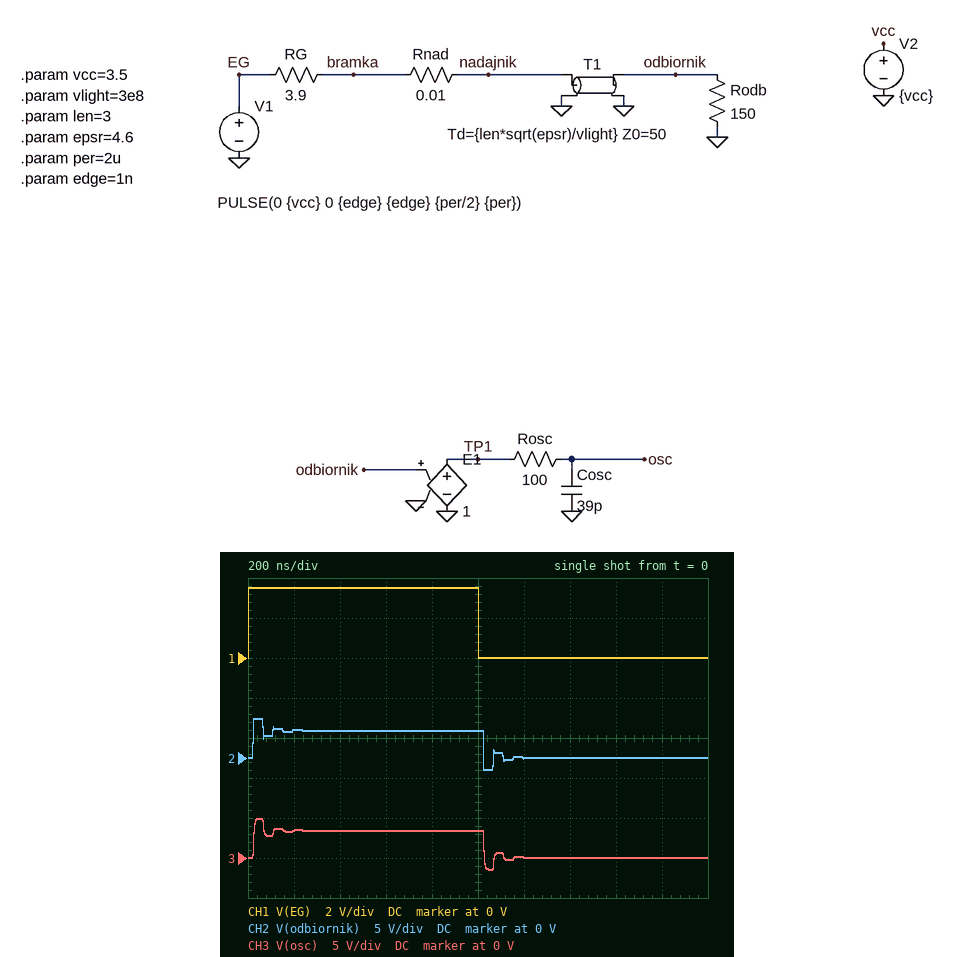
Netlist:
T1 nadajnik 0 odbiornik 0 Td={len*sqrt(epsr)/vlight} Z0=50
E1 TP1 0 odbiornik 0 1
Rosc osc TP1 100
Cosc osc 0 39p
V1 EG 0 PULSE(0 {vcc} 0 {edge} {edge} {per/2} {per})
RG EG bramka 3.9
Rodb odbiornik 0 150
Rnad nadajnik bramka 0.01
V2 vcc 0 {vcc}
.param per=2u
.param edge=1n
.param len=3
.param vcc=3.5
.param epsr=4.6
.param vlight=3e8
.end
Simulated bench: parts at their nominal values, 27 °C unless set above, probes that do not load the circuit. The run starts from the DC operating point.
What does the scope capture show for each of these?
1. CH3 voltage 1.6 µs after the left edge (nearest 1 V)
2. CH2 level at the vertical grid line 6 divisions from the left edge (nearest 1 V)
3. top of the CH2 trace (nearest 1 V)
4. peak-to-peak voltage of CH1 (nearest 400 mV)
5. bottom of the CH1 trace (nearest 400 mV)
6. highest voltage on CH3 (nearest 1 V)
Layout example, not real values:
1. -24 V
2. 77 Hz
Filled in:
1. 0 V
2. 0 V
3. 5 V
4. 3.6 V
5. 0 V
6. 5 V
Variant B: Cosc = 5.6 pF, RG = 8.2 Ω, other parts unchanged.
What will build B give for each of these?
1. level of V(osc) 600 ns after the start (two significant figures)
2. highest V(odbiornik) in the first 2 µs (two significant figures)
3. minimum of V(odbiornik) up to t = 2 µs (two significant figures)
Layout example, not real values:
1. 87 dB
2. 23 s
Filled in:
1. 3.3 V
2. 4.5 V
3. -1.2 V
